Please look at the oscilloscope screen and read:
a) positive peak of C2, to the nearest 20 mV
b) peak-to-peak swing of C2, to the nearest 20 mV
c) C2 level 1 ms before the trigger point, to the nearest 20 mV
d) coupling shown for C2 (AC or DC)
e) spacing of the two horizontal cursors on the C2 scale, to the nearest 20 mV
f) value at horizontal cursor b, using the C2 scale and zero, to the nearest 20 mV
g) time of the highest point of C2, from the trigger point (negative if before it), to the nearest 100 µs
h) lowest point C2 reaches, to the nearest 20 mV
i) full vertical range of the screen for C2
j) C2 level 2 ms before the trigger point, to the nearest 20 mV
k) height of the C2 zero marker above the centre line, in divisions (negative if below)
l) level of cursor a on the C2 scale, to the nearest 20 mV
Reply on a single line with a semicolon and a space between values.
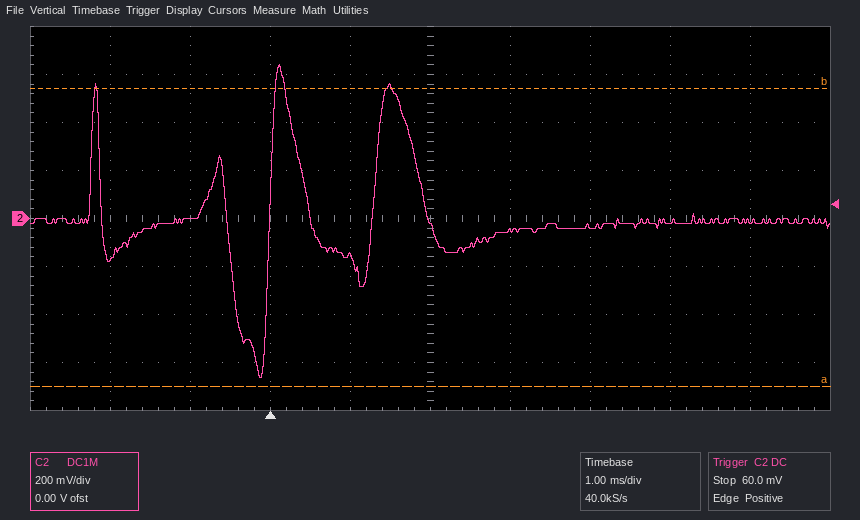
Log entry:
640 mV; 1.30 V; 0 mV; DC; 1.24 V; 540 mV; +100 µs; -660 mV; 1.6 V; -160 mV; 0.0 div; -700 mV
